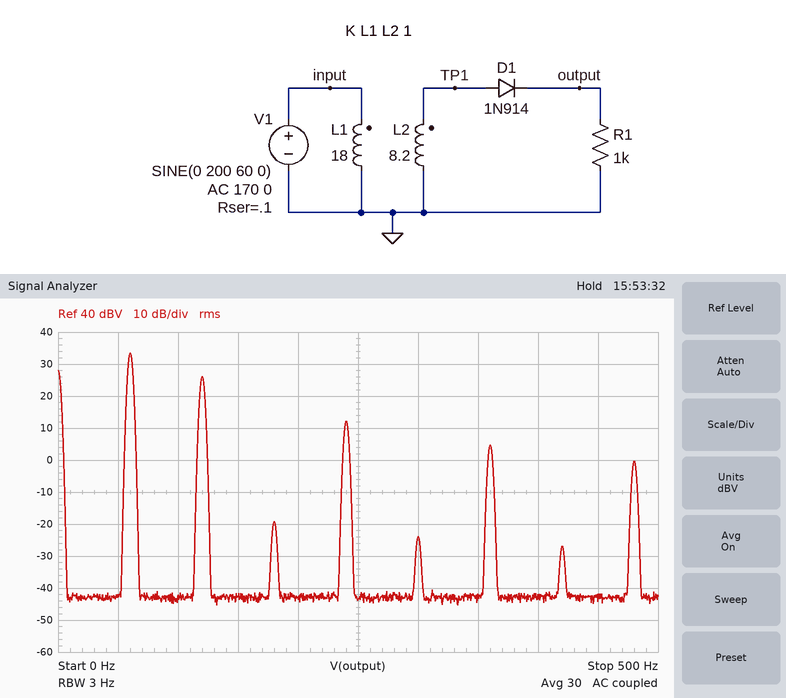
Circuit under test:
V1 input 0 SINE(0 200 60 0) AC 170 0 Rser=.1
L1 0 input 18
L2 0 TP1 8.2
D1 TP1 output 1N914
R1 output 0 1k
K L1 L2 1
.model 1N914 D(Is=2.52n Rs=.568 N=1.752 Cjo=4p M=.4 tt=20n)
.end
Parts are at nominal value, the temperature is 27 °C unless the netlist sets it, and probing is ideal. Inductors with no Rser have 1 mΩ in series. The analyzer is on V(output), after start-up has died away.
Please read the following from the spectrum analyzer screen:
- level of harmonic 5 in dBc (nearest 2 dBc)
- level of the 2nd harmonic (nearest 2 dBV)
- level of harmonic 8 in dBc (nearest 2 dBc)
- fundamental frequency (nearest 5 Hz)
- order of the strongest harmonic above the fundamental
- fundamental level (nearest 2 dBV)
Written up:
-58 dBc
26 dBV
-34 dBc
60 Hz
2
34 dBV
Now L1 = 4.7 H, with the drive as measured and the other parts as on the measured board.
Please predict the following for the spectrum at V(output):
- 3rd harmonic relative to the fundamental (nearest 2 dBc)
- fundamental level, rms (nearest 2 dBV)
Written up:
-58 dBc
40 dBV
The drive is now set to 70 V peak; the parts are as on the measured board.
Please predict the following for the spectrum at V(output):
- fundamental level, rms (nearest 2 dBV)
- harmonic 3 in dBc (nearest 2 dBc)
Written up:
24 dBV
-44 dBc
